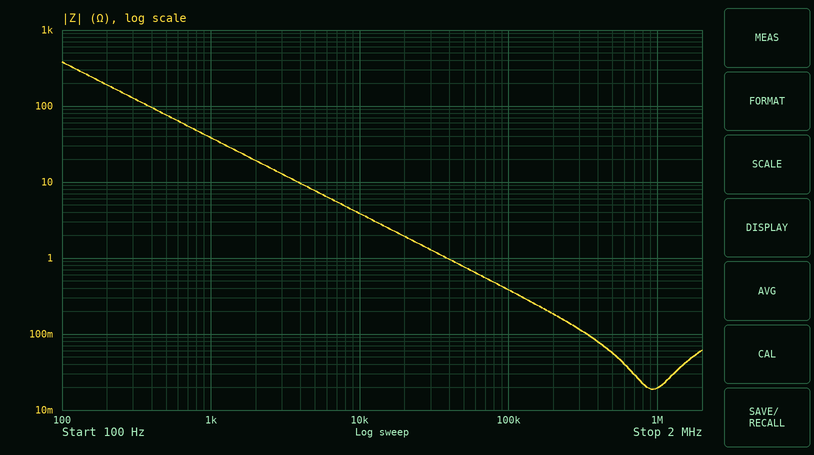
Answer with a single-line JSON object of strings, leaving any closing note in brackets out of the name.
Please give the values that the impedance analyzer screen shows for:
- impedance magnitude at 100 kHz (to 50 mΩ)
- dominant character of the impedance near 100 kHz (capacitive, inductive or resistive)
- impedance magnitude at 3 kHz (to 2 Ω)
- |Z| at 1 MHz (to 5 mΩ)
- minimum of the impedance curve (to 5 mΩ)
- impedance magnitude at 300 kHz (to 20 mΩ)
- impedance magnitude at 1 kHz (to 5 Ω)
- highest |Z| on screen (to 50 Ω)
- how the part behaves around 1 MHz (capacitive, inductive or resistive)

{"impedance magnitude at 100 kHz": "400 mΩ", "dominant character of the impedance near 100 kHz": "capacitive", "impedance magnitude at 3 kHz": "12 Ω", "|Z| at 1 MHz": "20 mΩ", "minimum of the impedance curve": "20 mΩ", "impedance magnitude at 300 kHz": "120 mΩ", "impedance magnitude at 1 kHz": "40 Ω", "highest |Z| on screen": "400 Ω", "how the part behaves around 1 MHz": "resistive"}
